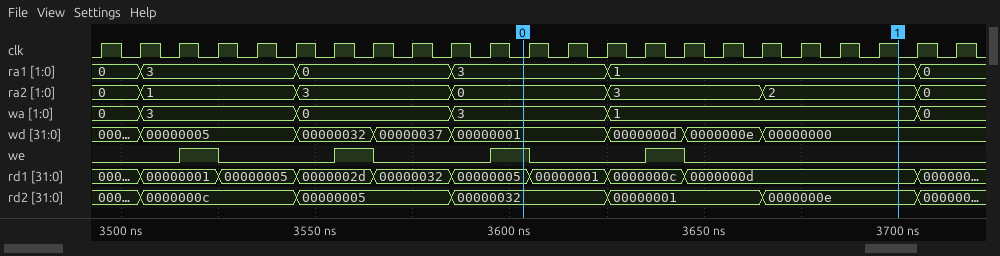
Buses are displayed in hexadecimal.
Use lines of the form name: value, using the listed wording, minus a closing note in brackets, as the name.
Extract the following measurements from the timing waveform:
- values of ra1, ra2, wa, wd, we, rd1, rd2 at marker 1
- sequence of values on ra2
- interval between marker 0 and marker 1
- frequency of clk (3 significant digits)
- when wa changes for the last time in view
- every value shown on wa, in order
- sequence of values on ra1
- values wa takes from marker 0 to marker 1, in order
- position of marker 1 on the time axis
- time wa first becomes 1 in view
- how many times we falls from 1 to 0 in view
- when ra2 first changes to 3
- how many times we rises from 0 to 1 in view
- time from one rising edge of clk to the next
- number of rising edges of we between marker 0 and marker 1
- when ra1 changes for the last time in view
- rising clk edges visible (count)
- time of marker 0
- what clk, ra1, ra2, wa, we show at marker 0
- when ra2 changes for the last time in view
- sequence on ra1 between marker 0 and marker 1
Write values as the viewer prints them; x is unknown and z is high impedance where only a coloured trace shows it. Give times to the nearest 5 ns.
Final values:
values of ra1, ra2, wa, wd, we, rd1, rd2 at marker 1: ra1=1, ra2=2, wa=1, wd=00000000, we=0, rd1=0000000d, rd2=0000000e
sequence of values on ra2: 0, 1, 3, 0, 3, 2, 0
interval between marker 0 and marker 1: 95 ns
frequency of clk: 100 MHz
when wa changes for the last time in view: 3705 ns
every value shown on wa, in order: 0, 3, 0, 3, 1, 0
sequence of values on ra1: 0, 3, 0, 3, 1, 0
values wa takes from marker 0 to marker 1, in order: 3, 1
position of marker 1 on the time axis: 3700 ns
time wa first becomes 1 in view: 3625 ns
how many times we falls from 1 to 0 in view: 4
when ra2 first changes to 3: 3545 ns
how many times we rises from 0 to 1 in view: 4
time from one rising edge of clk to the next: 10 ns
number of rising edges of we between marker 0 and marker 1: 1
when ra1 changes for the last time in view: 3705 ns
rising clk edges visible: 23
time of marker 0: 3605 ns
what clk, ra1, ra2, wa, we show at marker 0: clk=0, ra1=3, ra2=0, wa=3, we=1
when ra2 changes for the last time in view: 3705 ns
sequence on ra1 between marker 0 and marker 1: 3, 1
